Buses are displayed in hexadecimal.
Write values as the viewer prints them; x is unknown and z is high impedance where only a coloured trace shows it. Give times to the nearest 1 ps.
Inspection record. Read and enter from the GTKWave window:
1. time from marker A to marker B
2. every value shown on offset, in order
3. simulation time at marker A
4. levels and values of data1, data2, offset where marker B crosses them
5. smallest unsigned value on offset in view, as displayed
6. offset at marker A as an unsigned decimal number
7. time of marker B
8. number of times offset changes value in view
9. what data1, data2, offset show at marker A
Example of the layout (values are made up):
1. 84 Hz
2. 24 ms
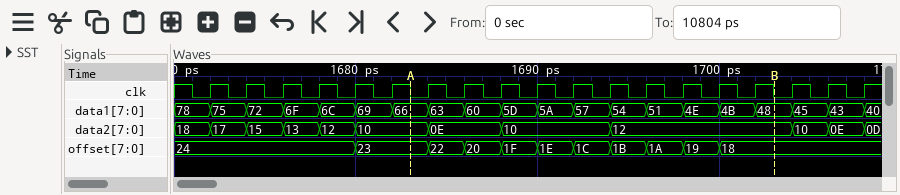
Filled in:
1. 20 ps
2. 24, 23, 22, 20, 1F, 1E, 1C, 1B, 1A, 19, 18
3. 1683 ps
4. data1=48, data2=12, offset=18
5. 18
6. 35
7. 1703 ps
8. 10
9. data1=66, data2=10, offset=23
